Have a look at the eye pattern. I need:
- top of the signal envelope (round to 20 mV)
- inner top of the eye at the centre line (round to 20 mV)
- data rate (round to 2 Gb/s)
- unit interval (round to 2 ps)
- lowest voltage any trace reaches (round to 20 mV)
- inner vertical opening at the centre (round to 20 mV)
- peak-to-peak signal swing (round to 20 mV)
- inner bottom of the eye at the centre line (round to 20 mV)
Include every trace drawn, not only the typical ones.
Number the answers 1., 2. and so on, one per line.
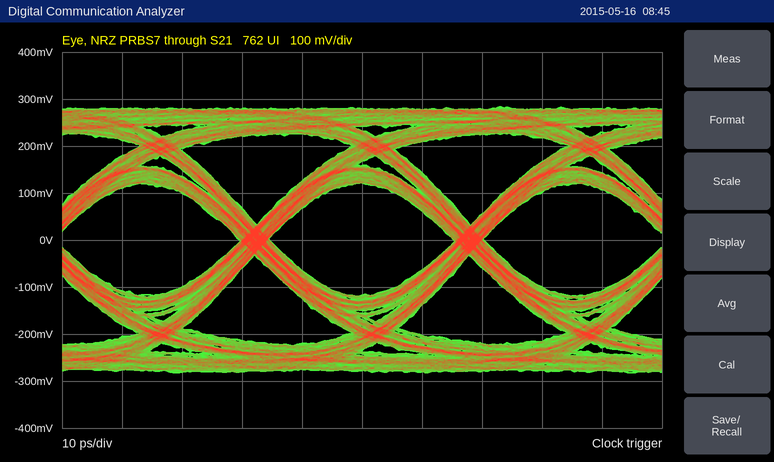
1. 280 mV
2. 120 mV
3. 28 Gb/s
4. 36 ps
5. -280 mV
6. 240 mV
7. 560 mV
8. -120 mV
